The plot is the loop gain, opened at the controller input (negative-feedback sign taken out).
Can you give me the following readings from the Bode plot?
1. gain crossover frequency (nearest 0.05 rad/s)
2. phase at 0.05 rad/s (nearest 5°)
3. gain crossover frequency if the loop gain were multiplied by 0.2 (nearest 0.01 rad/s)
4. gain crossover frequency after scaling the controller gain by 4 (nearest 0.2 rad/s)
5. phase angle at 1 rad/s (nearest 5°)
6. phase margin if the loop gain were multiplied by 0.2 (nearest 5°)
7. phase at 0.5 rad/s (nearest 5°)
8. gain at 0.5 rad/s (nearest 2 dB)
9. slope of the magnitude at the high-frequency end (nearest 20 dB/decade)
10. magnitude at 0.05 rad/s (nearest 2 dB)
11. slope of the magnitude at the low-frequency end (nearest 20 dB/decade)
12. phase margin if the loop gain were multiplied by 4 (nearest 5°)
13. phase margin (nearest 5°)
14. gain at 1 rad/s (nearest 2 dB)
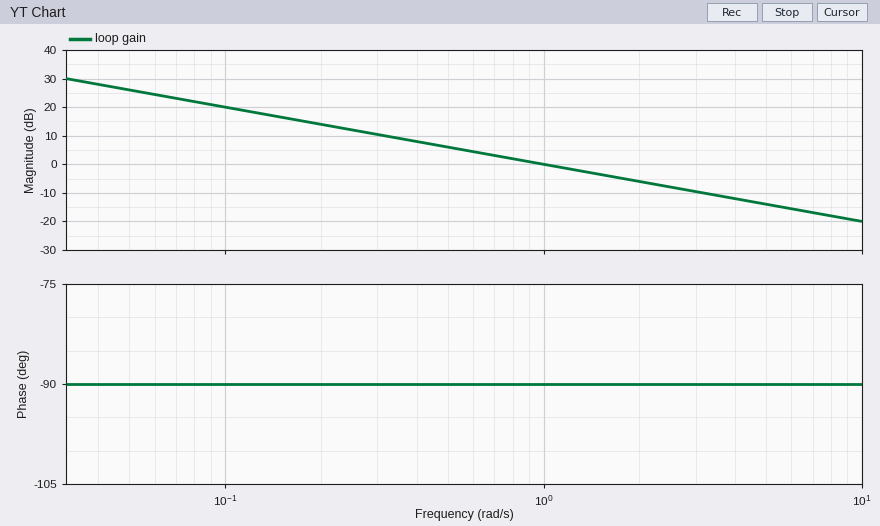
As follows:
1.00 rad/s
-90°
0.20 rad/s
4.0 rad/s
-90°
90°
-90°
6 dB
-20 dB/decade
26 dB
-20 dB/decade
90°
90°
0 dB
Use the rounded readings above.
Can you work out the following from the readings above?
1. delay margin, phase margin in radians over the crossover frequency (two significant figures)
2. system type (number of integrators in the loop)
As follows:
1.6 s
1
